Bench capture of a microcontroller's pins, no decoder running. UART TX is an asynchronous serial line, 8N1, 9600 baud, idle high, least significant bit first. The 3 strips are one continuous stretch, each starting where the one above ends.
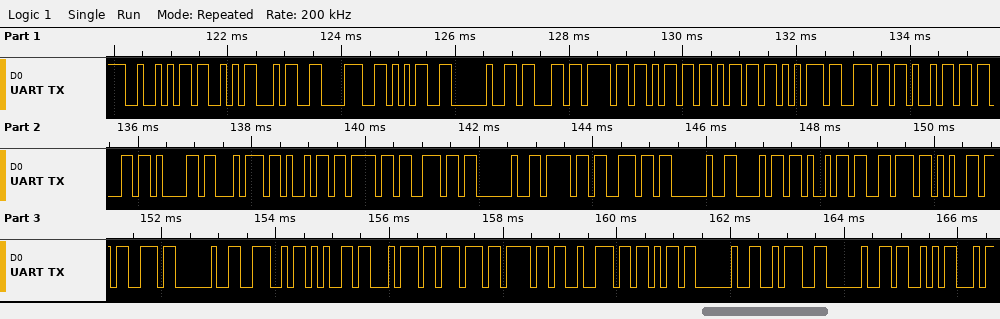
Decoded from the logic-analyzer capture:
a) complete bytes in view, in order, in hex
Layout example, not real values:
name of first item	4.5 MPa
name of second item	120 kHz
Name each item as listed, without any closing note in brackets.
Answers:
complete bytes in view, in order, in hex	52 53 34 38 35 20 63 6F 6D 6D 75 6E 69 63 61 74 69 6F 6E 20 6F 6E 20 68 69 76 65 73 20 4E 65 74 77 6F 72 6B 20 3A 20 53
